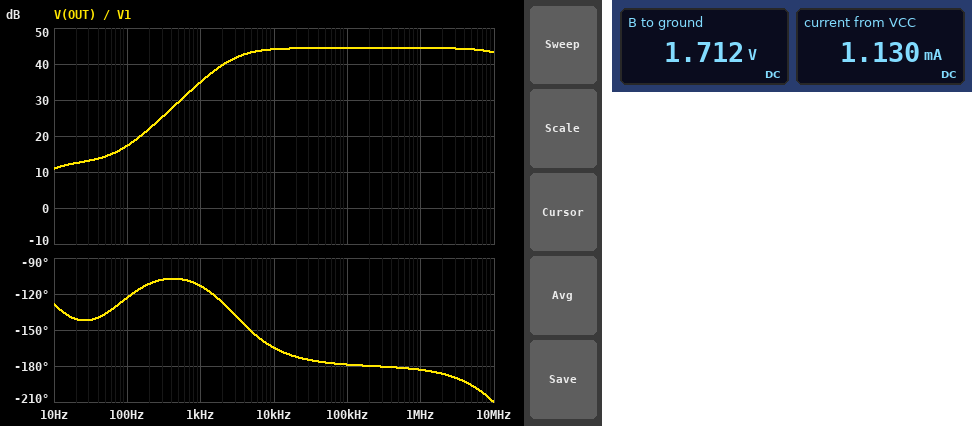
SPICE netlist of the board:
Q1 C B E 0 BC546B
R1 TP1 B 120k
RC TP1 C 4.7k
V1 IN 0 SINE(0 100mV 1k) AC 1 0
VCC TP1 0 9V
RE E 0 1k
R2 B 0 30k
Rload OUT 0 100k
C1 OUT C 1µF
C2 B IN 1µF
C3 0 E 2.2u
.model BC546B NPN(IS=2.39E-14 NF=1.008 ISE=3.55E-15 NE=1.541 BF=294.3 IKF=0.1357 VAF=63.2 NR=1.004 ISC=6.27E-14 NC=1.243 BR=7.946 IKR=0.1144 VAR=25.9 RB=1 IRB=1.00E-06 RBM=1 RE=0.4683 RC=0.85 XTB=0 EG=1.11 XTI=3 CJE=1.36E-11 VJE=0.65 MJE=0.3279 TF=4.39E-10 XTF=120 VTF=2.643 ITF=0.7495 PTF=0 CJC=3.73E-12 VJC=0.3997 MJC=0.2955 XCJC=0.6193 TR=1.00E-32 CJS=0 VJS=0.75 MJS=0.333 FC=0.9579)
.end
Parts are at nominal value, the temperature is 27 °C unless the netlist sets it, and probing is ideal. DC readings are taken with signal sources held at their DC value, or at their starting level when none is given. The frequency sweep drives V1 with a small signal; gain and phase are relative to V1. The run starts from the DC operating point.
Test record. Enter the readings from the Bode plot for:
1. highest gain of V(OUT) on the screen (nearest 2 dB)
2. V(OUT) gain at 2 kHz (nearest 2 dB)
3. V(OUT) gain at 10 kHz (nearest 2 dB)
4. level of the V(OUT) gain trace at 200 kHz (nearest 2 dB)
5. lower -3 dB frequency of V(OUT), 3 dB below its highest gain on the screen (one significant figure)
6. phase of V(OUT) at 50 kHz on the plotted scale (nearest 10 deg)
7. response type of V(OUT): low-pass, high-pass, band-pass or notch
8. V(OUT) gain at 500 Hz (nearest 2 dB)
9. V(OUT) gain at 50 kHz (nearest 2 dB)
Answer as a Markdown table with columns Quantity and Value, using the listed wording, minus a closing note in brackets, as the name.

| Quantity | Value |
|---|---|
| highest gain of V(OUT) on the screen | 44 dB |
| V(OUT) gain at 2 kHz | 40 dB |
| V(OUT) gain at 10 kHz | 44 dB |
| level of the V(OUT) gain trace at 200 kHz | 44 dB |
| lower -3 dB frequency of V(OUT), 3 dB below its highest gain on the screen | 3 kHz |
| phase of V(OUT) at 50 kHz on the plotted scale | -180 deg |
| response type of V(OUT): low-pass, high-pass, band-pass or notch | high-pass |
| V(OUT) gain at 500 Hz | 30 dB |
| V(OUT) gain at 50 kHz | 44 dB |
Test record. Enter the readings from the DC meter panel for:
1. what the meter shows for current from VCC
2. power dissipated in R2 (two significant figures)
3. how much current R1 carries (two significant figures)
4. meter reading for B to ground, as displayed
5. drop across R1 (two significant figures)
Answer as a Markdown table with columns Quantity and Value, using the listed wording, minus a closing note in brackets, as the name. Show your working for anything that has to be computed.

| Quantity | Value |
|---|---|
| what the meter shows for current from VCC | 1.130 mA |
| power dissipated in R2 | (1.712 V)^2 / 30 kΩ = 98 µW |
| how much current R1 carries | (9 V - 1.712 V) / 120 kΩ = 61 µA |
| meter reading for B to ground, as displayed | 1.712 V |
| drop across R1 | 9 V - 1.712 V = 7.3 V |
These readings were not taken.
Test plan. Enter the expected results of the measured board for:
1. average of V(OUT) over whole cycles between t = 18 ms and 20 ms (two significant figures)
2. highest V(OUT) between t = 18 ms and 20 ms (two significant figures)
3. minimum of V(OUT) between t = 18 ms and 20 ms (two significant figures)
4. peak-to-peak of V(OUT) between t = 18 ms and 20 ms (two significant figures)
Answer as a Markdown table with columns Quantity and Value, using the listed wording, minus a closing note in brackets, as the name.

| Quantity | Value |
|---|---|
| average of V(OUT) over whole cycles between t = 18 ms and 20 ms | 1.0 V |
| highest V(OUT) between t = 18 ms and 20 ms | 4.4 V |
| minimum of V(OUT) between t = 18 ms and 20 ms | -3.3 V |
| peak-to-peak of V(OUT) between t = 18 ms and 20 ms | 7.7 V |
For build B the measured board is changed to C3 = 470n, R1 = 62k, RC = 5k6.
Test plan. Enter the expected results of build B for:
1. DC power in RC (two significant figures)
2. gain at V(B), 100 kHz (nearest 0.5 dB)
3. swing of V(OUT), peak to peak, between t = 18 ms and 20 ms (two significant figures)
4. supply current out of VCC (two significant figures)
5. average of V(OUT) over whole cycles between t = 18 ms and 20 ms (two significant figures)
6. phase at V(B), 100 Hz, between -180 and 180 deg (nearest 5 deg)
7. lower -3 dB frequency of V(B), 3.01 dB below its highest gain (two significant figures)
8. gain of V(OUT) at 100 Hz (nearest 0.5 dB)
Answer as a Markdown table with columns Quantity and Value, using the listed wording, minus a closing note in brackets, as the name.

| Quantity | Value |
|---|---|
| DC power in RC | 10 mW |
| gain at V(B), 100 kHz | 0 dB |
| swing of V(OUT), peak to peak, between t = 18 ms and 20 ms | 2.0 V |
| supply current out of VCC | 1.5 mA |
| average of V(OUT) over whole cycles between t = 18 ms and 20 ms | 480 mV |
| phase at V(B), 100 Hz, between -180 and 180 deg | 50 deg |
| lower -3 dB frequency of V(B), 3.01 dB below its highest gain | 360 Hz |
| gain of V(OUT) at 100 Hz | -15.0 dB |
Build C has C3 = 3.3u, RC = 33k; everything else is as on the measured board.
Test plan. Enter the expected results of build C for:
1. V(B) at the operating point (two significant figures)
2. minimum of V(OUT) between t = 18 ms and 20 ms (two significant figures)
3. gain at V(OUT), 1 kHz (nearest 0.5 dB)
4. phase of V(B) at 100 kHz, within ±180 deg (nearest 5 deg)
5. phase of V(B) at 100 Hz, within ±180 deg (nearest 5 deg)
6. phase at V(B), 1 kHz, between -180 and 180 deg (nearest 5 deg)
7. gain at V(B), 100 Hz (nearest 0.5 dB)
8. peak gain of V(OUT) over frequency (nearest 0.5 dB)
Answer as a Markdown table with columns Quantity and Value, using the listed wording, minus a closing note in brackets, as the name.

| Quantity | Value |
|---|---|
| V(B) at the operating point | 920 mV |
| minimum of V(OUT) between t = 18 ms and 20 ms | -740 mV |
| gain at V(OUT), 1 kHz | -1.0 dB |
| phase of V(B) at 100 kHz, within ±180 deg | 0 deg |
| phase of V(B) at 100 Hz, within ±180 deg | 40 deg |
| phase at V(B), 1 kHz, between -180 and 180 deg | 20 deg |
| gain at V(B), 100 Hz | -9.5 dB |
| peak gain of V(OUT) over frequency | 0.5 dB |
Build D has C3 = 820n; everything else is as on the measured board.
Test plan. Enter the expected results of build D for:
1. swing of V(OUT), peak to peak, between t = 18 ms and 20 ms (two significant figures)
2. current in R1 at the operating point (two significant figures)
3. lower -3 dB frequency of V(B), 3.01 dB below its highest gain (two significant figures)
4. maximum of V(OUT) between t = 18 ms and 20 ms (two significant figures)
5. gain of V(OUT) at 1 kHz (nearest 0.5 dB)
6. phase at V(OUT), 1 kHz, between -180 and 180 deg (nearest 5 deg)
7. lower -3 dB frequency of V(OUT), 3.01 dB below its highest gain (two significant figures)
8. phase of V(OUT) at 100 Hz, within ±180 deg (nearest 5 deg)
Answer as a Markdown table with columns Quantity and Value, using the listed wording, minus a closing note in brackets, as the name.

| Quantity | Value |
|---|---|
| swing of V(OUT), peak to peak, between t = 18 ms and 20 ms | 4.5 V |
| current in R1 at the operating point | 61 µA |
| lower -3 dB frequency of V(B), 3.01 dB below its highest gain | 7.2 Hz |
| maximum of V(OUT) between t = 18 ms and 20 ms | 2.2 V |
| gain of V(OUT) at 1 kHz | 27.0 dB |
| phase at V(OUT), 1 kHz, between -180 and 180 deg | -110 deg |
| lower -3 dB frequency of V(OUT), 3.01 dB below its highest gain | 7.4 kHz |
| phase of V(OUT) at 100 Hz, within ±180 deg | -150 deg |
